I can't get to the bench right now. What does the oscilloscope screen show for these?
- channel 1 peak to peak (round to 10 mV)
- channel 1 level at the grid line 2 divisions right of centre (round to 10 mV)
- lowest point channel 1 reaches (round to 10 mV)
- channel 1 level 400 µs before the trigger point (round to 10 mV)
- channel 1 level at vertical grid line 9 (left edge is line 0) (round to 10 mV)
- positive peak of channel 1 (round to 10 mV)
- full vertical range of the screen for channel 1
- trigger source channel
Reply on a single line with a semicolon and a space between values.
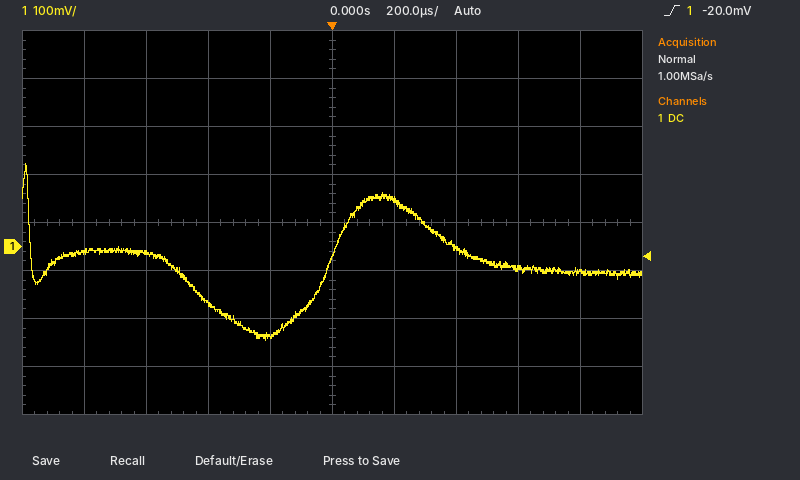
370 mV; 0 mV; -200 mV; -120 mV; -50 mV; 170 mV; 800 mV; channel 1
